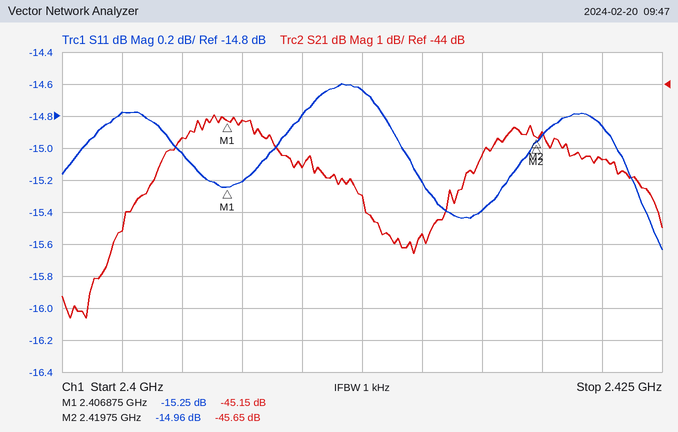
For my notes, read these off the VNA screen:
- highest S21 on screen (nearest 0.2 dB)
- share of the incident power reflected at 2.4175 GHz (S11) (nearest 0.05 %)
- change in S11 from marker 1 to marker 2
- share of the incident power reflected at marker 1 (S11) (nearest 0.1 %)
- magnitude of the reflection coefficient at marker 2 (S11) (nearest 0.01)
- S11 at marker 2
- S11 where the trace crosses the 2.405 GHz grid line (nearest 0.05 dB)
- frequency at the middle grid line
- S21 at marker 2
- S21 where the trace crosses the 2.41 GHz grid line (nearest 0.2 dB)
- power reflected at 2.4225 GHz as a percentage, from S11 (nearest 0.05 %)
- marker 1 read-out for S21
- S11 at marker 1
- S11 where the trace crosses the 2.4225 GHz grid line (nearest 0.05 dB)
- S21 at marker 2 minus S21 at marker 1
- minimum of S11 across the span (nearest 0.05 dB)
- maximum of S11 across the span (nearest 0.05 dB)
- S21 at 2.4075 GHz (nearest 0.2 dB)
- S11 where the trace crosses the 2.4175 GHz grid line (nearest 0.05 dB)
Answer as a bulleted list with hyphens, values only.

- -45.0 dB
- 2.90 %
- 0.29 dB
- 3.0 %
- 0.18
- -14.96 dB
- -15.05 dB
- 2.4125 GHz
- -45.65 dB
- -46.6 dB
- 3.25 %
- -45.15 dB
- -15.25 dB
- -14.85 dB
- -0.50 dB
- -15.65 dB
- -14.60 dB
- -45.2 dB
- -15.40 dB
